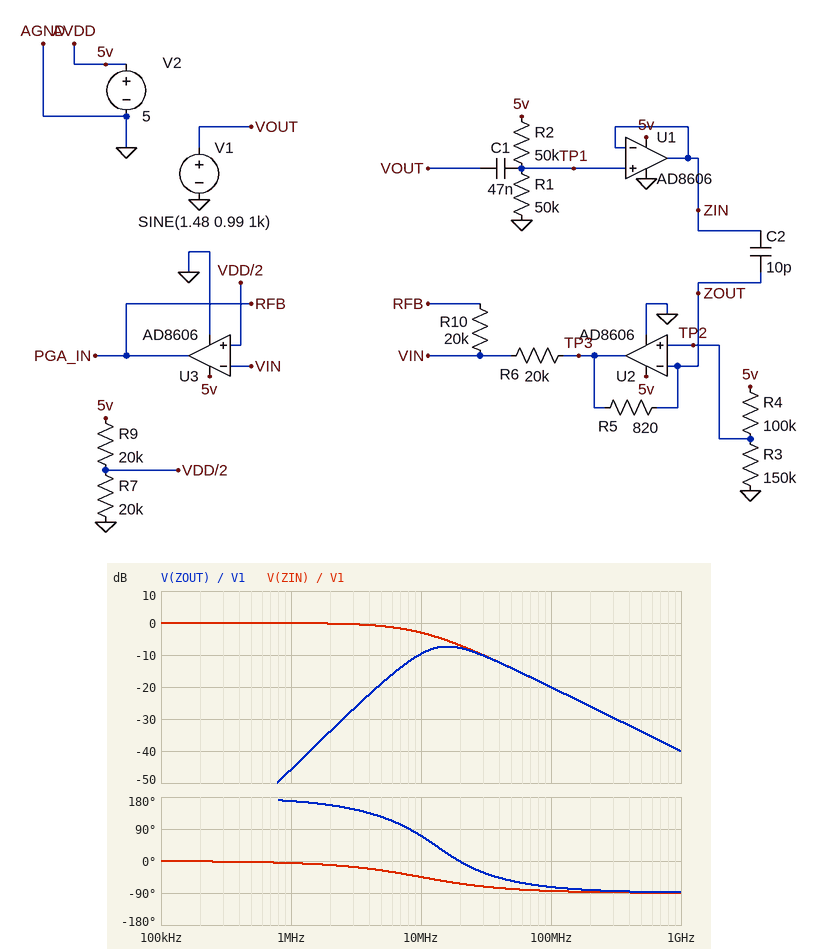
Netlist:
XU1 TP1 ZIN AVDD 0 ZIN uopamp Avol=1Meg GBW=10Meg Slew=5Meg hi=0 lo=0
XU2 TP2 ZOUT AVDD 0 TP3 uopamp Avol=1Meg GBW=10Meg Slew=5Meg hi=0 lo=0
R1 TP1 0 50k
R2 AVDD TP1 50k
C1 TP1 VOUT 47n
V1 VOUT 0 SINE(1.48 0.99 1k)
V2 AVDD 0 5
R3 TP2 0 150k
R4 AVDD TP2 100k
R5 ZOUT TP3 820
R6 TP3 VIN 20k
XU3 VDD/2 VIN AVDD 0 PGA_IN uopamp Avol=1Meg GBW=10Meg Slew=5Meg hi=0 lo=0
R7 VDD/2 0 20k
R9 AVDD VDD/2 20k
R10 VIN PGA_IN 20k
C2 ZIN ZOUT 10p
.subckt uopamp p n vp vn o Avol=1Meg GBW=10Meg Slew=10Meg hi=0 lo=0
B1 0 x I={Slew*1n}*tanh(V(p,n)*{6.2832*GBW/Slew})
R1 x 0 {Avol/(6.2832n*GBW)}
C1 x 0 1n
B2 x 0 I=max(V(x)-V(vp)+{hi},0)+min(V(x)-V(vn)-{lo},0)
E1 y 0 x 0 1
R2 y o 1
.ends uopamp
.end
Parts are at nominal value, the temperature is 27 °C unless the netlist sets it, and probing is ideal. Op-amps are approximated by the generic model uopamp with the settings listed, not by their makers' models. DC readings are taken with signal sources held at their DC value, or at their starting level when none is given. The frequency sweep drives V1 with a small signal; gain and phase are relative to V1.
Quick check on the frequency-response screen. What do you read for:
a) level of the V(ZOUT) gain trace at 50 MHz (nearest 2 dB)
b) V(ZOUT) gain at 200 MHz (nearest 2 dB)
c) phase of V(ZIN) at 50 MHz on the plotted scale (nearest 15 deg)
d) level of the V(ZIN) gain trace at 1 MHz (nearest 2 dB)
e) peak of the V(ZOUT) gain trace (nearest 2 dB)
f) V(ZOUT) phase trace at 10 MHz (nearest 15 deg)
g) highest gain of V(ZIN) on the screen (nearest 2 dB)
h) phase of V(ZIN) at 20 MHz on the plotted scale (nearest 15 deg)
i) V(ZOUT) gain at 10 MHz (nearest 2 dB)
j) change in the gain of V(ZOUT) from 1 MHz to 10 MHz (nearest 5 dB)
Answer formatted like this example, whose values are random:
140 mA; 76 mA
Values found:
-14 dB; -26 dB; -75 deg; 0 dB; -8 dB; 75 deg; 0 dB; -60 deg; -10 dB; 35 dB
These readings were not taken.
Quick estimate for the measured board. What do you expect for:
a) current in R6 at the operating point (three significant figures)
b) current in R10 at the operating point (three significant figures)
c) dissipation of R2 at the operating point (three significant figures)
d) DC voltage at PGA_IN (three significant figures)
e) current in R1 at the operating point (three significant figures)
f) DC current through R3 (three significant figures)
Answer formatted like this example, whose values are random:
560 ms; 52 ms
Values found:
25.0 µA; 25.0 µA; 125 µW; 2.00 V; 50.0 µA; 20.0 µA
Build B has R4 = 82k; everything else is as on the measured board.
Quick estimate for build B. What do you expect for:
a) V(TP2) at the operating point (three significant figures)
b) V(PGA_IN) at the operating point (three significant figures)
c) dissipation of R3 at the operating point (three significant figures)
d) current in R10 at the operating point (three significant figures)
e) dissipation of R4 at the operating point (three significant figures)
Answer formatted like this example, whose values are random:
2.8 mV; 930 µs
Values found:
3.23 V; 1.77 V; 69.7 µW; 36.6 µA; 38.1 µW
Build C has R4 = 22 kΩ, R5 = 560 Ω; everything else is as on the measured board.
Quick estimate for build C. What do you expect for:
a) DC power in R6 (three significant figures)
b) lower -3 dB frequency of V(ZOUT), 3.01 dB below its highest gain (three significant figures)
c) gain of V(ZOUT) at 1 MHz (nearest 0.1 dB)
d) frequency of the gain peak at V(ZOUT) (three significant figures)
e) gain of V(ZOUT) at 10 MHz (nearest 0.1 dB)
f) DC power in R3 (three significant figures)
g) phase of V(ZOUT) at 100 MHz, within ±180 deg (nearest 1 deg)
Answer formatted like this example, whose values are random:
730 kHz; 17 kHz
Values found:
173 µW; 10.4 MHz; -49.1 dB; 19.5 MHz; -13.6 dB; 127 µW; -68 deg
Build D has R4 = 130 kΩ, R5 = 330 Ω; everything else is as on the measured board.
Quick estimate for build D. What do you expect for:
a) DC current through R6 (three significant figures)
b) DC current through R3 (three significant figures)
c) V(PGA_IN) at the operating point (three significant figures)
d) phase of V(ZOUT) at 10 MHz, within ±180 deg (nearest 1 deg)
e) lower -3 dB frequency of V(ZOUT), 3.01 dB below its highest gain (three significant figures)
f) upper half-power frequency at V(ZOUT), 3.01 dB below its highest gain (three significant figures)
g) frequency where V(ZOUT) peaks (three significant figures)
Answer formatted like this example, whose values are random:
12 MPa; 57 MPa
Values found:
8.93 µA; 17.9 µA; 2.32 V; 83 deg; 11.8 MHz; 62.2 MHz; 25.7 MHz
